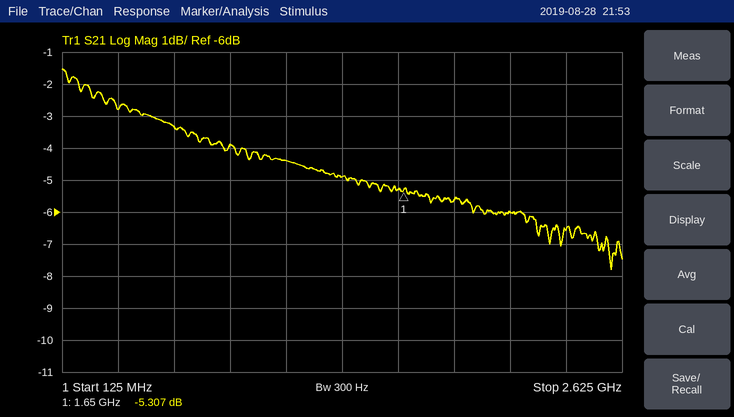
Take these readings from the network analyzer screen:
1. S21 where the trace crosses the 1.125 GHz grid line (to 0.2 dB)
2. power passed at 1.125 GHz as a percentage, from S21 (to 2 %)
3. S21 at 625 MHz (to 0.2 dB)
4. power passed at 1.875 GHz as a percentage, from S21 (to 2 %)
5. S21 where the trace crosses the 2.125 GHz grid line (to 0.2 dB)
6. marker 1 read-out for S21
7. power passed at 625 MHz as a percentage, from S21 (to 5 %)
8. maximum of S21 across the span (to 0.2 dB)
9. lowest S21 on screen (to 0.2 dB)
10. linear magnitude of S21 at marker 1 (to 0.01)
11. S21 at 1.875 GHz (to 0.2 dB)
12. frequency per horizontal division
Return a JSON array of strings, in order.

["-4.4 dB", "36 %", "-3.4 dB", "28 %", "-6.0 dB", "-5.307 dB", "45 %", "-1.6 dB", "-7.8 dB", "0.54", "-5.6 dB", "250 MHz"]
